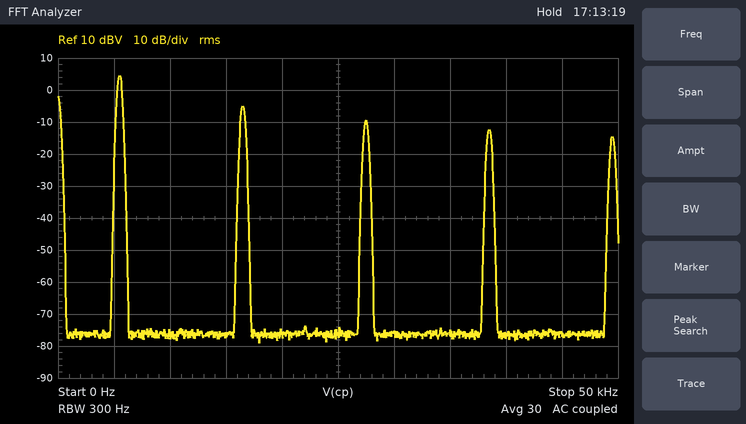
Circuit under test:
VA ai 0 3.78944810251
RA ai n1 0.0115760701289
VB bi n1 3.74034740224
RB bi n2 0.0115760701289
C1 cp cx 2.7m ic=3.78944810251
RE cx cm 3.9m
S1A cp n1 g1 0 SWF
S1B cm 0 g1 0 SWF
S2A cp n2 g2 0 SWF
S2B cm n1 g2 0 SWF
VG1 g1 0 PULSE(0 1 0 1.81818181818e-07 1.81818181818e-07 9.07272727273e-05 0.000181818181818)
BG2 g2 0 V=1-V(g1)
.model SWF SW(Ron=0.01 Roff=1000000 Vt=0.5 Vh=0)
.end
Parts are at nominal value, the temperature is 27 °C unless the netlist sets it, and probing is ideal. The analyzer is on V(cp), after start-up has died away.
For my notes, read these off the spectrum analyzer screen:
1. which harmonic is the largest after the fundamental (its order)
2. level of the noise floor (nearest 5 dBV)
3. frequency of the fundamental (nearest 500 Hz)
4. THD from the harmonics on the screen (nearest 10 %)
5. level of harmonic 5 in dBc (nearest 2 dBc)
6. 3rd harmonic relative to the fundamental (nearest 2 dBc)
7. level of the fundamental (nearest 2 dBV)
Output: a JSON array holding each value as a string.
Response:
["3", "-75 dBV", "5.5 kHz", "40 %", "-14 dBc", "-10 dBc", "4 dBV"]
